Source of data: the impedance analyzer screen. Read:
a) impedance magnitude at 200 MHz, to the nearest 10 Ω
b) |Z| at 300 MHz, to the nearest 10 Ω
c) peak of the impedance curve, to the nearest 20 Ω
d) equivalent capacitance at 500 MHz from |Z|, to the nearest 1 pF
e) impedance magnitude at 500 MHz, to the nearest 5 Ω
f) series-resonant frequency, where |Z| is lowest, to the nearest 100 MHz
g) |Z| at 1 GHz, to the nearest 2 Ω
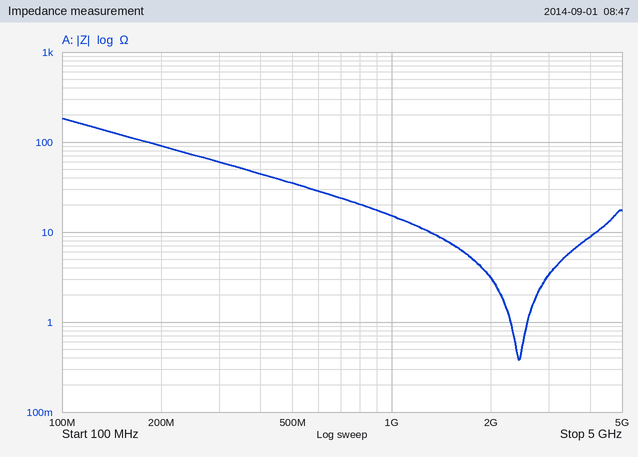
90 Ω
60 Ω
180 Ω
9 pF
35 Ω
2.4 GHz
16 Ω
